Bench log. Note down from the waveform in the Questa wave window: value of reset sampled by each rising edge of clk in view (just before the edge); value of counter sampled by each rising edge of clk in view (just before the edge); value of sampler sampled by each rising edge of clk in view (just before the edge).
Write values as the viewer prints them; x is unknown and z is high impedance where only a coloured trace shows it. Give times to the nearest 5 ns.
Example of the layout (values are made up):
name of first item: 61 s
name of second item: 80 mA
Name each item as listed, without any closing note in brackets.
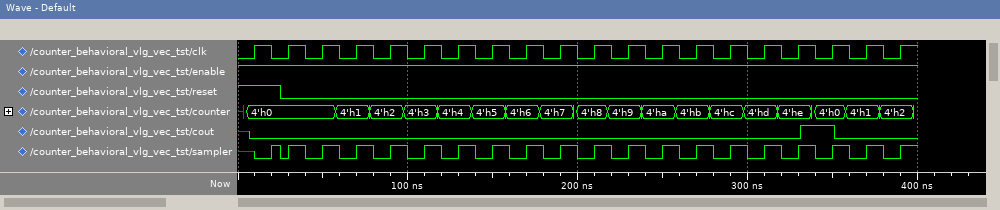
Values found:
value of reset sampled by each rising edge of clk in view: 1 0 0 0 0 0 0 0 0 0 0 0 0 0 0 0 0 0 0 0
value of counter sampled by each rising edge of clk in view: 4'h0, 4'h0, 4'h0, 4'h1, 4'h2, 4'h3, 4'h4, 4'h5, 4'h6, 4'h7, 4'h8, 4'h9, 4'ha, 4'hb, 4'hc, 4'hd, 4'he, 4'h0, 4'h1, 4'h2
value of sampler sampled by each rising edge of clk in view: x 0 0 0 0 0 0 0 0 0 0 0 0 0 0 0 0 0 0 0
